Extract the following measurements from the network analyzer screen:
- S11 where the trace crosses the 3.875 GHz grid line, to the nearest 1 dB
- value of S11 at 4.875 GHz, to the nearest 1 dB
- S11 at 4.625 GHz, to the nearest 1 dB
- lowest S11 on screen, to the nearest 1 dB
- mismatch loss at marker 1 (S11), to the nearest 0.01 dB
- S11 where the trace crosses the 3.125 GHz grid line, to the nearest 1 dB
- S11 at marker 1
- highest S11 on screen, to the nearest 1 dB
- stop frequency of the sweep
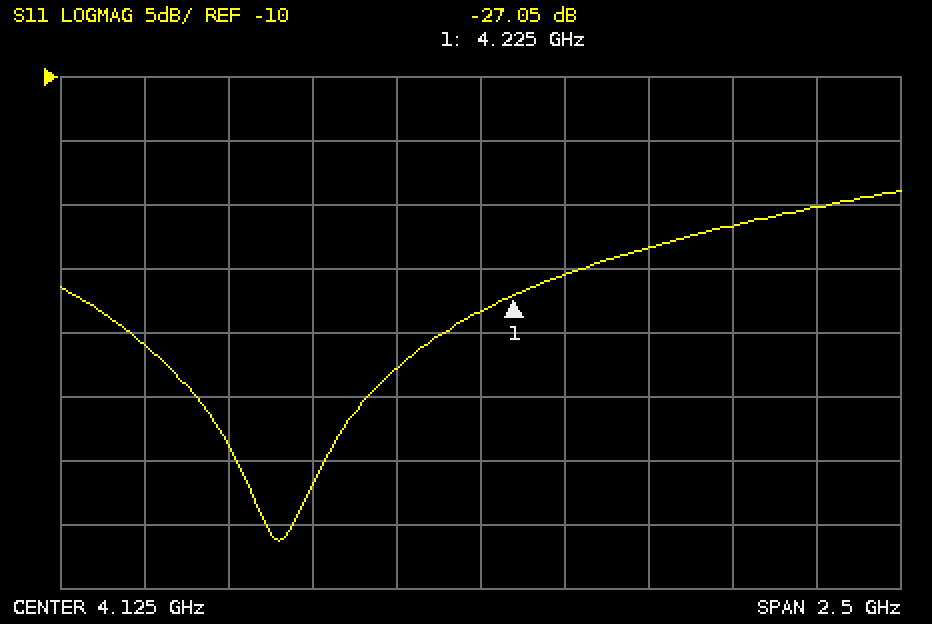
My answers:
-33 dB
-22 dB
-23 dB
-46 dB
0.01 dB
-31 dB
-27.05 dB
-19 dB
5.375 GHz
